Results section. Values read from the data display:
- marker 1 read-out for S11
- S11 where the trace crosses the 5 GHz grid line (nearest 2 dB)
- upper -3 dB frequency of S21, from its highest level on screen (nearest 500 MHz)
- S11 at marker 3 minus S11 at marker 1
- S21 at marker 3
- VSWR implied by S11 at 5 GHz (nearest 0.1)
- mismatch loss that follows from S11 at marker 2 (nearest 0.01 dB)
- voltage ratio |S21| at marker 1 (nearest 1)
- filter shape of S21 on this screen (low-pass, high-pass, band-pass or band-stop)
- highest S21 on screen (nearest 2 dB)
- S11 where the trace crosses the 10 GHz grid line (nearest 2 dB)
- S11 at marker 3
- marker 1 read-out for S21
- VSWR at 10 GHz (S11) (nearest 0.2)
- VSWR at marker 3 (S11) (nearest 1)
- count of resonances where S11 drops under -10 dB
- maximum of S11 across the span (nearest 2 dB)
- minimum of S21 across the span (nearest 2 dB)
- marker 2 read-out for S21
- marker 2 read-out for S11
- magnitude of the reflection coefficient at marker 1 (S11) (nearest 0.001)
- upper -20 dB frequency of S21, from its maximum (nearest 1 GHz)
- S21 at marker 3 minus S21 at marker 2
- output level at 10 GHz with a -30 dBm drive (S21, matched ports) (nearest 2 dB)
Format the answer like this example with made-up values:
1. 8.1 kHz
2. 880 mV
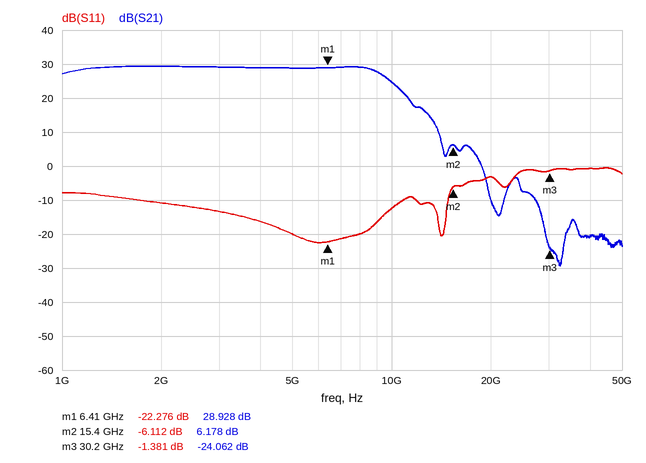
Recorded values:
1. -22.276 dB
2. -20 dB
3. 9.5 GHz
4. 20.895 dB
5. -24.062 dB
6. 1.2
7. 1.22 dB
8. 28
9. low-pass
10. 30 dB
11. -12 dB
12. -1.381 dB
13. 28.928 dB
14. 1.6
15. 13
16. 2
17. 0 dB
18. -30 dB
19. 6.178 dB
20. -6.112 dB
21. 0.077
22. 14 GHz
23. -30.240 dB
24. -6 dBm
